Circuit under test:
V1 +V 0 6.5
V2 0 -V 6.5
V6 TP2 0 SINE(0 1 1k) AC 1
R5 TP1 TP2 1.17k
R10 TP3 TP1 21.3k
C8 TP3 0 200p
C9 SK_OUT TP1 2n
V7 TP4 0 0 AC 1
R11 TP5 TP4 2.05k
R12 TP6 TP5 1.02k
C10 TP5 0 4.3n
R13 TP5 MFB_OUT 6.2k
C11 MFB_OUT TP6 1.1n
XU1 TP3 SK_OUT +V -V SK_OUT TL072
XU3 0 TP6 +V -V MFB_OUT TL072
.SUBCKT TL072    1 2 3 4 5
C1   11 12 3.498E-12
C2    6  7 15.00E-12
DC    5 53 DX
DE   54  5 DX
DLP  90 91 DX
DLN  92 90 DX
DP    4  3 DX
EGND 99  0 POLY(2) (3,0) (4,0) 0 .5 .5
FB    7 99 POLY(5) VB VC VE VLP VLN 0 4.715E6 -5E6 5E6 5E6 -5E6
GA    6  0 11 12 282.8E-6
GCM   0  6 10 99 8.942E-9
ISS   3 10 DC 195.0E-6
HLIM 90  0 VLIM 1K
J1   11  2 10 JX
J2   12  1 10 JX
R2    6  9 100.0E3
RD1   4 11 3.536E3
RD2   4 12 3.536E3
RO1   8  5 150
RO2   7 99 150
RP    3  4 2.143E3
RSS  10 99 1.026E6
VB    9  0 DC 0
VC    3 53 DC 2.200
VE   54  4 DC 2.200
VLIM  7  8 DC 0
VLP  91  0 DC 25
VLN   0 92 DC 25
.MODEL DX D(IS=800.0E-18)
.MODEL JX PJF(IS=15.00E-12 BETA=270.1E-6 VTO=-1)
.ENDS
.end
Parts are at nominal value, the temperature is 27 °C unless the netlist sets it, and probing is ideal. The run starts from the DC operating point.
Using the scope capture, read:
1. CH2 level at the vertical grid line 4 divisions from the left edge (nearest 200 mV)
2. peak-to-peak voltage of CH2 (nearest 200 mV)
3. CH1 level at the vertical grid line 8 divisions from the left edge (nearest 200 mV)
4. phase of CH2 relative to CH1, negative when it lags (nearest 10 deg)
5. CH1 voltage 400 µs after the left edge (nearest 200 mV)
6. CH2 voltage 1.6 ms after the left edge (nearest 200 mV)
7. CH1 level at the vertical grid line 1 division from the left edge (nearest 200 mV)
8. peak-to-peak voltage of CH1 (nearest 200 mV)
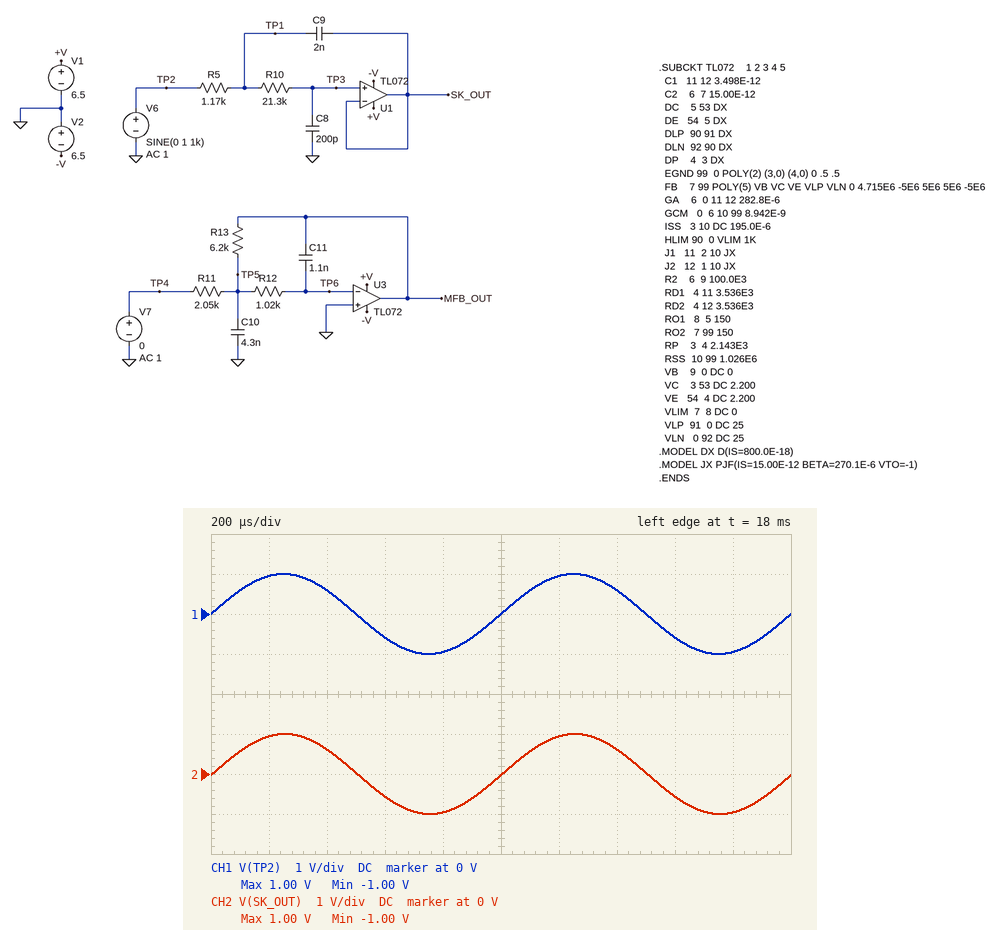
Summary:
-1.0 V
2.0 V
-600 mV
0 deg
600 mV
-600 mV
1.0 V
2.0 V
